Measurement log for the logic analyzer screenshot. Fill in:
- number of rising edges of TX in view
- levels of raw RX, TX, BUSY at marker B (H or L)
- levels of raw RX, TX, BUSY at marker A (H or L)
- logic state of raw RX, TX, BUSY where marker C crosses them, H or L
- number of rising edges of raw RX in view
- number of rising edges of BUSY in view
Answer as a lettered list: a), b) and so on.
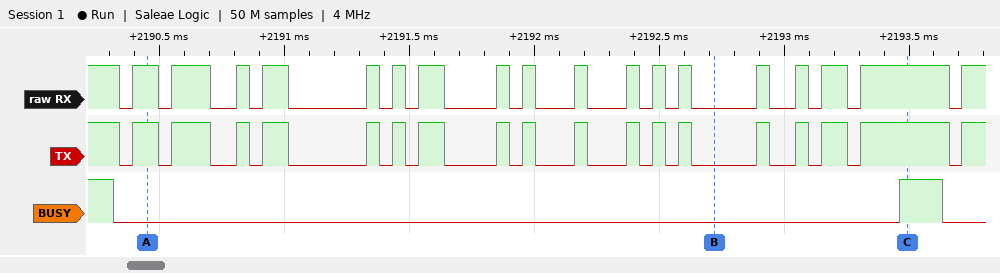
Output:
a) 18
b) raw RX=L, TX=L, BUSY=L
c) raw RX=H, TX=H, BUSY=L
d) raw RX=H, TX=H, BUSY=H
e) 18
f) 1
